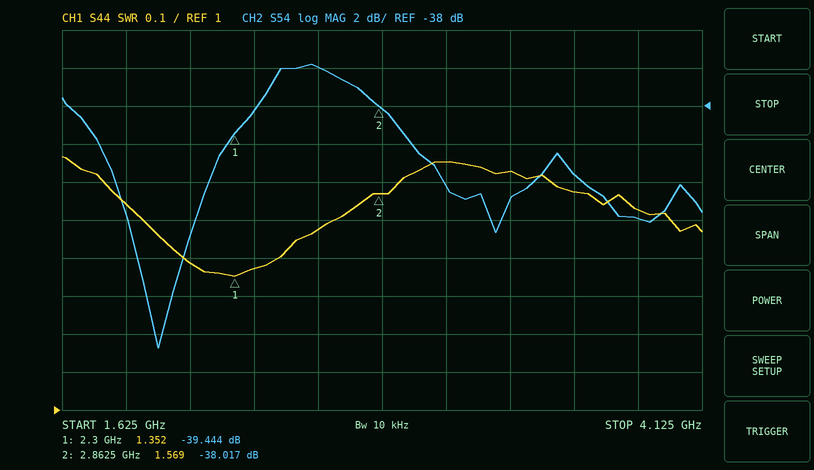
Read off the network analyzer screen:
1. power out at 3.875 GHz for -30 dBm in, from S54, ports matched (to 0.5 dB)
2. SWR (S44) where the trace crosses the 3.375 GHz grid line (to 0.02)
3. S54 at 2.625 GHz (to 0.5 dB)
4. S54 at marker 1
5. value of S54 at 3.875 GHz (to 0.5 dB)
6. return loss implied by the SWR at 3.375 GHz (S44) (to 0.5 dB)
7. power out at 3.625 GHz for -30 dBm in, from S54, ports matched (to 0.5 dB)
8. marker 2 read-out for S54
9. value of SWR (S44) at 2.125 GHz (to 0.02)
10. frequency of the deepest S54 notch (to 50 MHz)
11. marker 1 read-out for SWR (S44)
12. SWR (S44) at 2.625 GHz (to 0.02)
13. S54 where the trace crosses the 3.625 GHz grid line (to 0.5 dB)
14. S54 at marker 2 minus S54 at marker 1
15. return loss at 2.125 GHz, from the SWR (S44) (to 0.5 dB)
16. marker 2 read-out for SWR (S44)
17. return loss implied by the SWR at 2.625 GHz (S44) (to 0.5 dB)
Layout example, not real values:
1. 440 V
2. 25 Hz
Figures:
1. -74.0 dBm
2. 1.62
3. -36.0 dB
4. -39.444 dB
5. -44.0 dB
6. 12.5 dB
7. -71.5 dBm
8. -38.017 dB
9. 1.38
10. 2.00 GHz
11. 1.352
12. 1.48
13. -41.5 dB
14. 1.427 dB
15. 16.0 dB
16. 1.569
17. 14.5 dB
